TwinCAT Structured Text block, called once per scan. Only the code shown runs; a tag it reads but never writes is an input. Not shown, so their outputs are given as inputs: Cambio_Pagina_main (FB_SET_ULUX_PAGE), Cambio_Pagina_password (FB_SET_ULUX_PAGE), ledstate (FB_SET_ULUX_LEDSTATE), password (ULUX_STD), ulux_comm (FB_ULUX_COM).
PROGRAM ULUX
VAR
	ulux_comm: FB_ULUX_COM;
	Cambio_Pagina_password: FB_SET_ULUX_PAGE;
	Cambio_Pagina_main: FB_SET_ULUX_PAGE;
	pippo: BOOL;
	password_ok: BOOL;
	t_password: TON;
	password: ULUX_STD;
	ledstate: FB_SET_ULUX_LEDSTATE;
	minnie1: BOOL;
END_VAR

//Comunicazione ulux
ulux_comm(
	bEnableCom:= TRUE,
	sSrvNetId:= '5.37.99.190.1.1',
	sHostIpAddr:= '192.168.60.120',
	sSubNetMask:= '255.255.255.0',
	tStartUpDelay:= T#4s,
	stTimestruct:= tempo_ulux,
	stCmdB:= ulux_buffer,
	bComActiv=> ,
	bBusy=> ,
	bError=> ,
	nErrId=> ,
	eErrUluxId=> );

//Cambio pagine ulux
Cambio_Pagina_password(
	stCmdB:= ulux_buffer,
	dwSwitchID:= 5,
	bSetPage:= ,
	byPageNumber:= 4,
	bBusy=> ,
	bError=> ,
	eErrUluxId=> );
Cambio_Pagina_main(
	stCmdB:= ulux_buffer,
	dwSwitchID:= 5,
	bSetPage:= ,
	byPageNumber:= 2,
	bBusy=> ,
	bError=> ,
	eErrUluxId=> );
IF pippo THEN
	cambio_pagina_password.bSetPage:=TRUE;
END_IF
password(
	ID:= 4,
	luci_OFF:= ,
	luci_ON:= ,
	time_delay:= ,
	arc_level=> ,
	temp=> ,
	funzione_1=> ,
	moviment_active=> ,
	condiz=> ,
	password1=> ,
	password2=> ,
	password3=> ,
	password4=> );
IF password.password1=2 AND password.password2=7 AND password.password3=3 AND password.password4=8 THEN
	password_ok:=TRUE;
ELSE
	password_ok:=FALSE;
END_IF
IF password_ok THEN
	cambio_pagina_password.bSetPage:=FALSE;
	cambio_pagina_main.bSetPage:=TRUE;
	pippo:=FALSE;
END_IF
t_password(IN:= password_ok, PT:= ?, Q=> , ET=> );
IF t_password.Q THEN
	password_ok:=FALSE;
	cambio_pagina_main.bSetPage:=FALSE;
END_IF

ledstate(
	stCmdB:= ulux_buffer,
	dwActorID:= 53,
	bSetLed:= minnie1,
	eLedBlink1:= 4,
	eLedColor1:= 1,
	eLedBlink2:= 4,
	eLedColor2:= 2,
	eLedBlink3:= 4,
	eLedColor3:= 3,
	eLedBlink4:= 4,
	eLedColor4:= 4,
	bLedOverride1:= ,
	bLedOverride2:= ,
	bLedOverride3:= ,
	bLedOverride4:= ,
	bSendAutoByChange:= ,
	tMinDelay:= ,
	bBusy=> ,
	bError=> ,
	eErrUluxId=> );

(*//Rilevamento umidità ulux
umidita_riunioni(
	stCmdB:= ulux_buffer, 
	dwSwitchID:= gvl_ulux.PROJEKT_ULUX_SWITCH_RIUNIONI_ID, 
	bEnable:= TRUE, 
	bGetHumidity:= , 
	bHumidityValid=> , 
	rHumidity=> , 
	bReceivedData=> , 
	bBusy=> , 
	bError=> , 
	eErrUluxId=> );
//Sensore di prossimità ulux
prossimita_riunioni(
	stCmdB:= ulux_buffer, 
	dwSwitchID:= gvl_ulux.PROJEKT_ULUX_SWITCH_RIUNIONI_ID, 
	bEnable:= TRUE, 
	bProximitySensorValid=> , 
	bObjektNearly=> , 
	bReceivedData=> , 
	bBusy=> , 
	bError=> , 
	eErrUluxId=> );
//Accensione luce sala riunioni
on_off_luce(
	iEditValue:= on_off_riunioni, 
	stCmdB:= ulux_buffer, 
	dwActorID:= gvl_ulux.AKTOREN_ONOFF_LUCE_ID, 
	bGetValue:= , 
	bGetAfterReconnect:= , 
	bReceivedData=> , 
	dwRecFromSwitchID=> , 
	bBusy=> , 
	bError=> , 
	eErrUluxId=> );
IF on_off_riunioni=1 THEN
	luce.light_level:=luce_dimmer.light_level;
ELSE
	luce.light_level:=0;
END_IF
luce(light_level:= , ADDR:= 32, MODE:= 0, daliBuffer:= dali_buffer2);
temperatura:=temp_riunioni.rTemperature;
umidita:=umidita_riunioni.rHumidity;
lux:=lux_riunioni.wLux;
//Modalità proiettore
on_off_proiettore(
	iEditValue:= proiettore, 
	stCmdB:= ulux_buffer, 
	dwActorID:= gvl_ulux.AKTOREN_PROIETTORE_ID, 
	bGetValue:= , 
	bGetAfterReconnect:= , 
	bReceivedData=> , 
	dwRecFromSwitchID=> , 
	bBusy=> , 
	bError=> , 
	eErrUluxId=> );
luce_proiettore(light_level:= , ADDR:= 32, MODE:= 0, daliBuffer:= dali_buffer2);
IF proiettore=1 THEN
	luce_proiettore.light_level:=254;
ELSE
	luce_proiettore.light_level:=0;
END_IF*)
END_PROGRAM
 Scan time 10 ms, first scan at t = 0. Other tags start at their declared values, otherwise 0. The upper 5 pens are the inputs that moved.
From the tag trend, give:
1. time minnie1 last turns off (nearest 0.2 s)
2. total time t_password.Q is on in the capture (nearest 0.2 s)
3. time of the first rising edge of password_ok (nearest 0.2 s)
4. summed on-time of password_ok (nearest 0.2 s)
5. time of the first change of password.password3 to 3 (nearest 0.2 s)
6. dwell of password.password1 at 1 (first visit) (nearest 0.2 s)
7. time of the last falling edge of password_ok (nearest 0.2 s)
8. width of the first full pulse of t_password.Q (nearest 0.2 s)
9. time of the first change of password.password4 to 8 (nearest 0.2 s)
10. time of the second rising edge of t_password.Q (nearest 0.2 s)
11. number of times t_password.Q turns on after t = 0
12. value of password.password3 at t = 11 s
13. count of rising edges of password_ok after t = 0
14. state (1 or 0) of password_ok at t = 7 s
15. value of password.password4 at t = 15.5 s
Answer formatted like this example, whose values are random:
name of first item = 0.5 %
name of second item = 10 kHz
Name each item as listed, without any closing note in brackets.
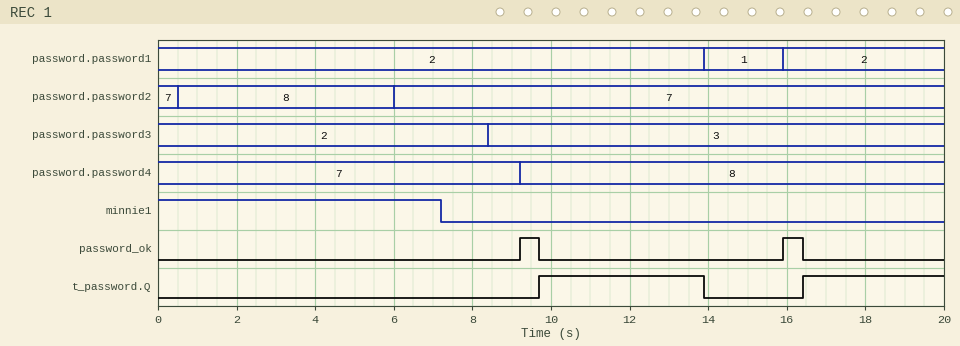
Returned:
time minnie1 last turns off = 7.2 s
total time t_password.Q is on in the capture = 7.8 s
time of the first rising edge of password_ok = 9.2 s
summed on-time of password_ok = 1.0 s
time of the first change of password.password3 to 3 = 8.4 s
dwell of password.password1 at 1 (first visit) = 2.0 s
time of the last falling edge of password_ok = 16.4 s
width of the first full pulse of t_password.Q = 4.2 s
time of the first change of password.password4 to 8 = 9.2 s
time of the second rising edge of t_password.Q = 16.4 s
number of times t_password.Q turns on after t = 0 = 2
value of password.password3 at t = 11 s = 3
count of rising edges of password_ok after t = 0 = 2
state (1 or 0) of password_ok at t = 7 s = 0
value of password.password4 at t = 15.5 s = 8
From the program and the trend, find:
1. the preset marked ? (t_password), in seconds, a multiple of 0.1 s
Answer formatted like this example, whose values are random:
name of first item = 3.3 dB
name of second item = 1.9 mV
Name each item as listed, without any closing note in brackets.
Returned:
the preset marked ? (t_password), in seconds, a multiple of 0.1 s = 0.5 s
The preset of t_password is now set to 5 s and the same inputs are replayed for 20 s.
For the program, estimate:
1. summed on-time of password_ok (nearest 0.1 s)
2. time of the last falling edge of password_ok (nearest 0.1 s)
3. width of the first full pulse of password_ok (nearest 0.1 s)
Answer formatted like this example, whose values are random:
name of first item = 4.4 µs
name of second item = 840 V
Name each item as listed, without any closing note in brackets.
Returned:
summed on-time of password_ok = 8.8 s
time of the last falling edge of password_ok = 13.9 s
width of the first full pulse of password_ok = 4.7 s
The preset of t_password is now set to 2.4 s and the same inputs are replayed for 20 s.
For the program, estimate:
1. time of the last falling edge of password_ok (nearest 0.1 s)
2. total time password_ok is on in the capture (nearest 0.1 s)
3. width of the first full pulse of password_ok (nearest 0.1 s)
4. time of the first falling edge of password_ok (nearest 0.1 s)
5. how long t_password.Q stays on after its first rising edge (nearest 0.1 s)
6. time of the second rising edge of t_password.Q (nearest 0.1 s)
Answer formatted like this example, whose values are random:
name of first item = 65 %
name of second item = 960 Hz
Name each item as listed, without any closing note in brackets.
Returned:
time of the last falling edge of password_ok = 18.3 s
total time password_ok is on in the capture = 4.8 s
width of the first full pulse of password_ok = 2.4 s
time of the first falling edge of password_ok = 11.6 s
how long t_password.Q stays on after its first rising edge = 2.3 s
time of the second rising edge of t_password.Q = 18.3 s
